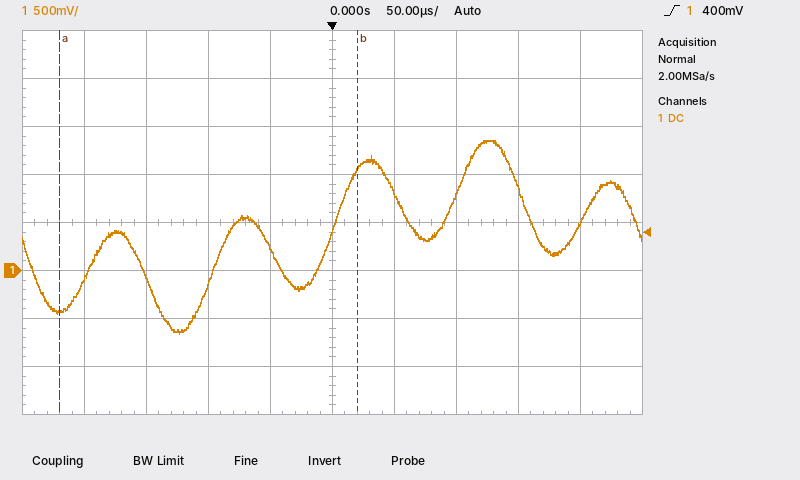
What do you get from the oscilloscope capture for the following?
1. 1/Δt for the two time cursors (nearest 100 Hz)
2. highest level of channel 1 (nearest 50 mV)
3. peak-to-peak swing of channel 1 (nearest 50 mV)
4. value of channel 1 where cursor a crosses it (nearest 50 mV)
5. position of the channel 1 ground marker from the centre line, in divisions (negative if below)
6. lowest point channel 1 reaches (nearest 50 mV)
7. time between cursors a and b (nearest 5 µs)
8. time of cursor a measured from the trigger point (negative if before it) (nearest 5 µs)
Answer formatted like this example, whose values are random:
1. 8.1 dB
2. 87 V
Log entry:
1. 4.2 kHz
2. 1.35 V
3. 2.00 V
4. -450 mV
5. -1.0 div
6. -650 mV
7. 240 µs
8. -220 µs
